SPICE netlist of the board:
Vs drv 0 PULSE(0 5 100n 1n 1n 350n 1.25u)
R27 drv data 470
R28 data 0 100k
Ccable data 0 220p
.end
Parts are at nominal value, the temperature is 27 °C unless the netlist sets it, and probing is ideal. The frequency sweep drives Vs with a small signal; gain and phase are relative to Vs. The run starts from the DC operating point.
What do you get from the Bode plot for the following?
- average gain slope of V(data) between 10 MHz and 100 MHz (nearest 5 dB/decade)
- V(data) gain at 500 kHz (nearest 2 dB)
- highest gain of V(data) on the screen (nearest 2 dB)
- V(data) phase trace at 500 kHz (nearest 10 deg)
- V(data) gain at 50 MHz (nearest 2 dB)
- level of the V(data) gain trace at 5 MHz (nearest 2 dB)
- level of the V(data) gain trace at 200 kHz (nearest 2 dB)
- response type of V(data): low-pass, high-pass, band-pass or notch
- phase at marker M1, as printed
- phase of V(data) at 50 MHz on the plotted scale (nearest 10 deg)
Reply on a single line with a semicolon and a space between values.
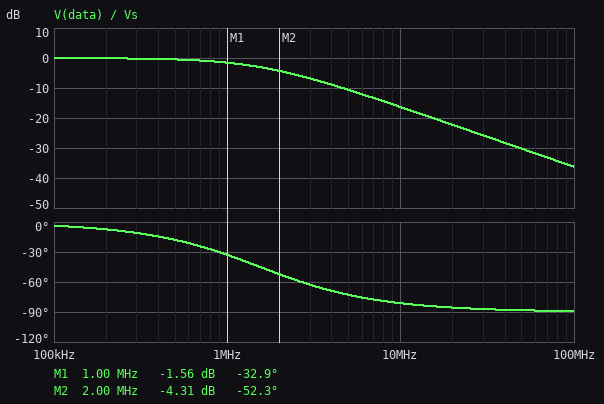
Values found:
-20 dB/decade; 0 dB; 0 dB; -20 deg; -30 dB; -10 dB; 0 dB; low-pass; -32.9 deg; -90 deg
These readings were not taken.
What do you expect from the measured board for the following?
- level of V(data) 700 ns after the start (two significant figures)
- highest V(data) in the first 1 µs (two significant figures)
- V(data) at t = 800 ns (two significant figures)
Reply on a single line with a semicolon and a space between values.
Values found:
430 mV; 4.8 V; 160 mV
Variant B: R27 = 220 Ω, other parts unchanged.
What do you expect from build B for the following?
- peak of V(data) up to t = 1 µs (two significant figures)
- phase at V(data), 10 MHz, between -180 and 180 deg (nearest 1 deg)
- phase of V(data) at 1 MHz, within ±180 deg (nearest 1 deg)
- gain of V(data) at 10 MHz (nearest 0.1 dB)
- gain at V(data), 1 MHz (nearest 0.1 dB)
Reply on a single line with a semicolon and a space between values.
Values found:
5.0 V; -72 deg; -17 deg; -10.1 dB; -0.4 dB
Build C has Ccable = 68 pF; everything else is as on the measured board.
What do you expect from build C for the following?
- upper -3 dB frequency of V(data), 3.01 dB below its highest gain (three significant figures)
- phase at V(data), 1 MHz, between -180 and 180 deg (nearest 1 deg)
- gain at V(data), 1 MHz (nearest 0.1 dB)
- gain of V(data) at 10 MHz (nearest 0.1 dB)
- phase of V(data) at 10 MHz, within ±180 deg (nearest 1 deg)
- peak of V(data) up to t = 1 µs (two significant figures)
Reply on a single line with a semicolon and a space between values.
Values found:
5.00 MHz; -11 deg; -0.2 dB; -7.0 dB; -63 deg; 5.0 V
